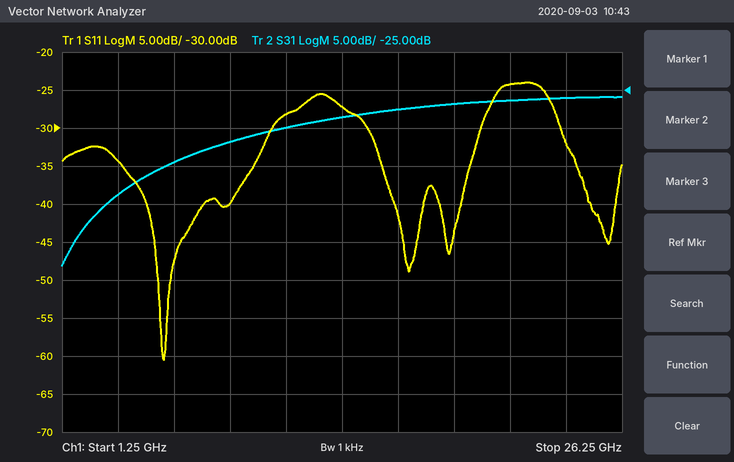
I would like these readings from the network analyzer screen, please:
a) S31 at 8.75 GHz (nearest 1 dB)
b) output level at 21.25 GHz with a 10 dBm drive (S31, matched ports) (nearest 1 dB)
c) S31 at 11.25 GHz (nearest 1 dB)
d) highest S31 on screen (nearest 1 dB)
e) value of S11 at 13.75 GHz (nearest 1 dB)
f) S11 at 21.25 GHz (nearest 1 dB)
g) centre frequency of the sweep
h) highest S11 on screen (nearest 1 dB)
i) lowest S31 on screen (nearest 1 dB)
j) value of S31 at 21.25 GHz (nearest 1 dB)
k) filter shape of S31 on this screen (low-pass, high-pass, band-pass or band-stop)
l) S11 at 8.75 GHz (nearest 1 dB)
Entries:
-32 dB
-16 dBm
-30 dB
-26 dB
-27 dB
-24 dB
13.75 GHz
-24 dB
-48 dB
-26 dB
high-pass
-40 dB
